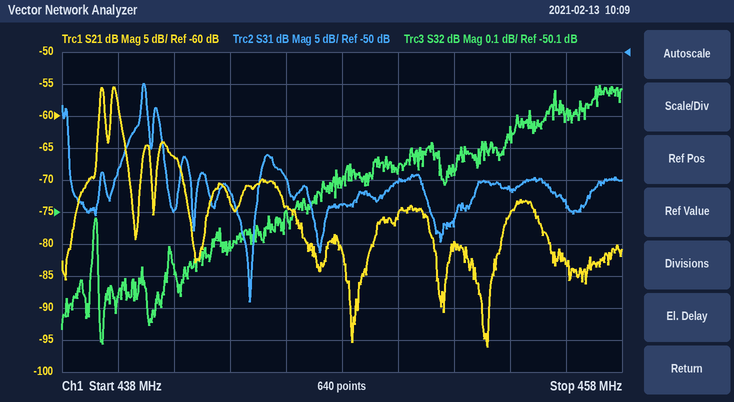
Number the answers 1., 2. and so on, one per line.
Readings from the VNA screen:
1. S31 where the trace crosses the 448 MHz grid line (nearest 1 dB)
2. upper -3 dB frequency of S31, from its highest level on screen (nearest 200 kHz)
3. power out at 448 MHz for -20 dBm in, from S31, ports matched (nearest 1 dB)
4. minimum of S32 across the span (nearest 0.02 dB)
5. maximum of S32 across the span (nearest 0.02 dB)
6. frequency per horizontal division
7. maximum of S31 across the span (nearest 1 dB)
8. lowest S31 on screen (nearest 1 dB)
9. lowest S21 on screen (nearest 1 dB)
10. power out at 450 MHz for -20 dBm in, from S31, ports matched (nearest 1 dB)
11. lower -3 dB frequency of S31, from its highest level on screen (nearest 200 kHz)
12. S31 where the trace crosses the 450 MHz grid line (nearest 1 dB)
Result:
1. -74 dB
2. 441.0 MHz
3. -94 dBm
4. -50.52 dB
5. -49.70 dB
6. 2 MHz
7. -55 dB
8. -89 dB
9. -96 dB
10. -90 dBm
11. 440.8 MHz
12. -70 dB
